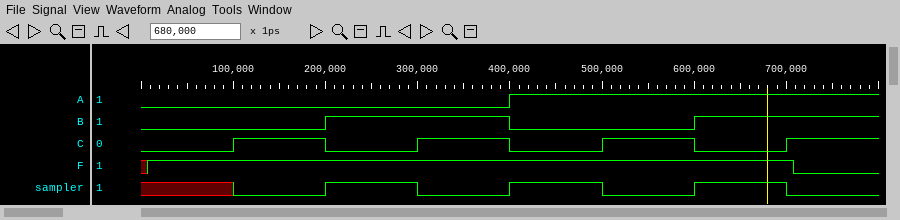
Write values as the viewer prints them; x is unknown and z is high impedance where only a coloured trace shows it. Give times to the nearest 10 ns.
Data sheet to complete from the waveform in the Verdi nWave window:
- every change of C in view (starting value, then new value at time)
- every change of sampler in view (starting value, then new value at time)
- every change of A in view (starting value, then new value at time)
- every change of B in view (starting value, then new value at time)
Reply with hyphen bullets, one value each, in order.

- 0, 1 at 100 ns, 0 at 200 ns, 1 at 300 ns, 0 at 400 ns, 1 at 500 ns, 0 at 600 ns, 1 at 700 ns
- x, 0 at 100 ns, 1 at 200 ns, 0 at 300 ns, 1 at 400 ns, 0 at 500 ns, 1 at 600 ns, 0 at 700 ns
- 0, 1 at 400 ns
- 0, 1 at 200 ns, 0 at 400 ns, 1 at 600 ns
